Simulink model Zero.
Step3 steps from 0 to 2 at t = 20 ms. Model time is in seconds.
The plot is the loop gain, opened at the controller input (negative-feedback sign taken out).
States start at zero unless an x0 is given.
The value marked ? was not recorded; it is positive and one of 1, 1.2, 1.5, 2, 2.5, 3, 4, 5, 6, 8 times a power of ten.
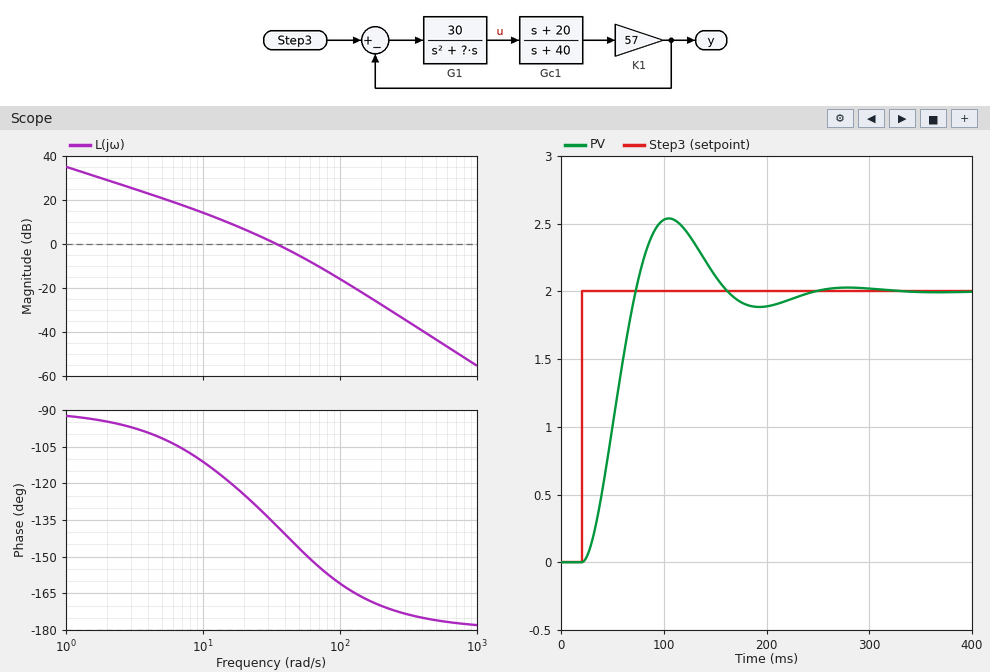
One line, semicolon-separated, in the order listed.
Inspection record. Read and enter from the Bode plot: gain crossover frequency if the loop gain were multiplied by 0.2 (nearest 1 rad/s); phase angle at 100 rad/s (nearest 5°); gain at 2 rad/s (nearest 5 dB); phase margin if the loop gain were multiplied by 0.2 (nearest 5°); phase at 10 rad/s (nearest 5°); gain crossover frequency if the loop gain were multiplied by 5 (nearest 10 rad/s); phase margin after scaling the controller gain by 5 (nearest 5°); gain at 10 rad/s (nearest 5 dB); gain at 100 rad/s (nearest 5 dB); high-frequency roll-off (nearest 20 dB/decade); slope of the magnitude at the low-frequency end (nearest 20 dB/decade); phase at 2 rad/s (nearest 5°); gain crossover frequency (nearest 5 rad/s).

10 rad/s; -160°; 30 dB; 70°; -110°; 90 rad/s; 20°; 15 dB; -15 dB; -40 dB/decade; -20 dB/decade; -95°; 35 rad/s
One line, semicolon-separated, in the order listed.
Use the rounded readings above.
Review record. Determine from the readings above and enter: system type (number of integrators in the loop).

1
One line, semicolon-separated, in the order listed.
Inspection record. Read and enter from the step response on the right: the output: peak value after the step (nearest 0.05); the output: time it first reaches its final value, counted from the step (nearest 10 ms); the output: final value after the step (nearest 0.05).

2.55; 50 ms; 2.00
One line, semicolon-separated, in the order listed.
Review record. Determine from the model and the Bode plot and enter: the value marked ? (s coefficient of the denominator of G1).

15
